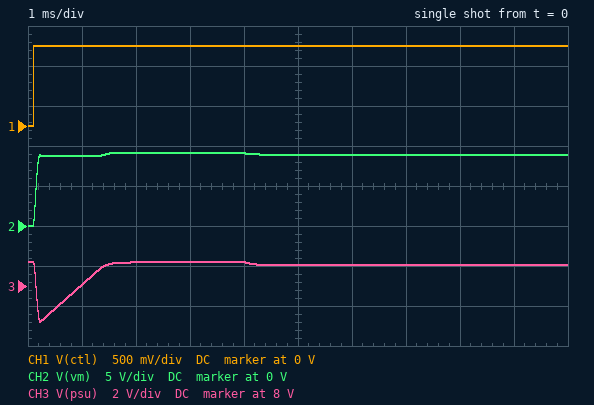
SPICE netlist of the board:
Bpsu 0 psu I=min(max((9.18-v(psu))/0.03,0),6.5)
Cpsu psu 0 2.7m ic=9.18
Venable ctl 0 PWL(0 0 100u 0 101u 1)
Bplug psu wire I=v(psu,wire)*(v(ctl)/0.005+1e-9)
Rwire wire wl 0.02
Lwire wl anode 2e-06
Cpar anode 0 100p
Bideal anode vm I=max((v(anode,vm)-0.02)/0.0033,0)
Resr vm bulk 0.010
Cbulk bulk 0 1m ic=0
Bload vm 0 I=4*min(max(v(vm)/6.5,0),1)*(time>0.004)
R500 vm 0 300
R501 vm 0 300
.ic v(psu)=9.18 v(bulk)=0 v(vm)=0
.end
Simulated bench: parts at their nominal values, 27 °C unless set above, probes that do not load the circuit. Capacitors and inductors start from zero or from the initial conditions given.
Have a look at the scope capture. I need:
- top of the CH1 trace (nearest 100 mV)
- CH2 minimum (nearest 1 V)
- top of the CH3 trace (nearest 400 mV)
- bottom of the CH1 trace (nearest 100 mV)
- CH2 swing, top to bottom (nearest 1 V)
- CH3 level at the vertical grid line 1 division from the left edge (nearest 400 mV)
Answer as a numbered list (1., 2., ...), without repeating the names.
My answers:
1. 1.0 V
2. 0 V
3. 9.2 V
4. 0 V
5. 9 V
6. 8.0 V
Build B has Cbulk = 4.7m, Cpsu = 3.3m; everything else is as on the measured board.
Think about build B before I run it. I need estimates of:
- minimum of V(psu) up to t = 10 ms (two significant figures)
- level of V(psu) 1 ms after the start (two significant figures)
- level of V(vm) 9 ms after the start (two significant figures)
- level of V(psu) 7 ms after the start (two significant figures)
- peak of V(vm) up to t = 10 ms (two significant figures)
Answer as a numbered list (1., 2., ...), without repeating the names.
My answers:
1. 3.6 V
2. 4.6 V
3. 8.4 V
4. 8.0 V
5. 8.7 V
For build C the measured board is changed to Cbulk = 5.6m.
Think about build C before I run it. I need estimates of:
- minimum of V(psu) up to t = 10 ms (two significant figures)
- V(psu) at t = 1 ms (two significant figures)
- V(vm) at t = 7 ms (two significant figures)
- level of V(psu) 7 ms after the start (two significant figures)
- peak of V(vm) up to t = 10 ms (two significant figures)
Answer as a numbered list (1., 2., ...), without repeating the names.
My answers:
1. 2.6 V
2. 3.8 V
3. 6.9 V
4. 7.1 V
5. 7.8 V
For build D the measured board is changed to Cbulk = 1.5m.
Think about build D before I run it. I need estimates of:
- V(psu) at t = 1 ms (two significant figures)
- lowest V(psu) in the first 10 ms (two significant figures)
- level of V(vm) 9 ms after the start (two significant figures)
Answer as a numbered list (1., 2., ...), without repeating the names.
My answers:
1. 7.2 V
2. 5.4 V
3. 8.9 V
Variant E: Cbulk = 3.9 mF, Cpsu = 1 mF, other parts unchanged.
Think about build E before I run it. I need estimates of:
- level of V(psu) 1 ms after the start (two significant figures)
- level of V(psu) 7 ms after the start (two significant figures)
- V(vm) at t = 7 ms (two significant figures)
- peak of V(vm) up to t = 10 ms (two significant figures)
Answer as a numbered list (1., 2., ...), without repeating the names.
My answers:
1. 3.2 V
2. 8.7 V
3. 8.5 V
4. 8.9 V
